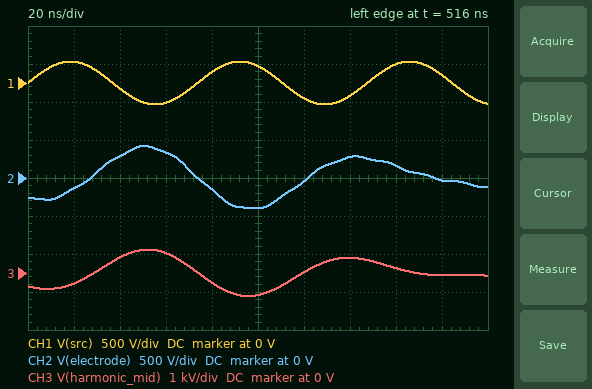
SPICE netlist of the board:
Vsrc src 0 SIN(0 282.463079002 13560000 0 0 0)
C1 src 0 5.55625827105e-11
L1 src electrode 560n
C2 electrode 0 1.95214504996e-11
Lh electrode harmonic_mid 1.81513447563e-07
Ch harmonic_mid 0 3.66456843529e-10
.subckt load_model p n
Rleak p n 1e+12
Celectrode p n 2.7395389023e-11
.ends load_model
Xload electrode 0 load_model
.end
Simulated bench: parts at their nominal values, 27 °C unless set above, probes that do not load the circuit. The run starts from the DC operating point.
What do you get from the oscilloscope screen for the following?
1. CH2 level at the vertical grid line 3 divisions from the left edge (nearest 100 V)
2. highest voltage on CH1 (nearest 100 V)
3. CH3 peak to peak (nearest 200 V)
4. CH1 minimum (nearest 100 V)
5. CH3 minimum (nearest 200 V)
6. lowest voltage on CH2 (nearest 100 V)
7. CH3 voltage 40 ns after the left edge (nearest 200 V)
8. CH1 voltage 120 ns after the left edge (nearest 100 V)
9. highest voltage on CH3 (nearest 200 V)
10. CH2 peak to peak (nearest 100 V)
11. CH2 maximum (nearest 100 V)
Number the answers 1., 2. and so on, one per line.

1. 300 V
2. 300 V
3. 1.2 kV
4. -300 V
5. -600 V
6. -400 V
7. 400 V
8. -200 V
9. 600 V
10. 800 V
11. 400 V
